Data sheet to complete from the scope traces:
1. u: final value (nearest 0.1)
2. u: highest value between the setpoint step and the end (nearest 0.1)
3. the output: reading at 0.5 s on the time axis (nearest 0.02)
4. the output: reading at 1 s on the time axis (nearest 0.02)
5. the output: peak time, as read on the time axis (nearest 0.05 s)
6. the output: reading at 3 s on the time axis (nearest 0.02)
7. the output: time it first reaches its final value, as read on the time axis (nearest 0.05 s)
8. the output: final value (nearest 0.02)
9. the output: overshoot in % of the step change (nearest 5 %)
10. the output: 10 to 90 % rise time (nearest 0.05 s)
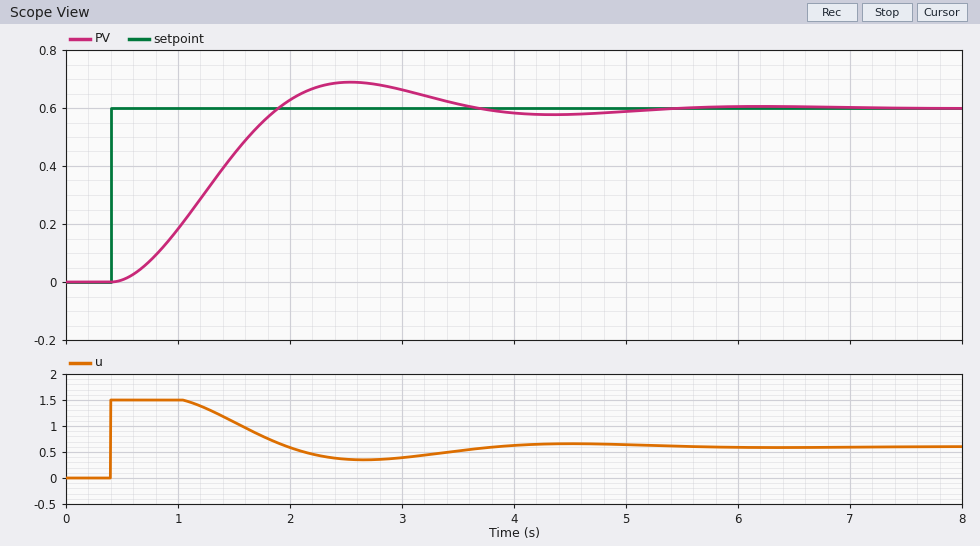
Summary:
0.6
1.5
0.00
0.18
2.55 s
0.66
1.90 s
0.60
15 %
1.00 s
